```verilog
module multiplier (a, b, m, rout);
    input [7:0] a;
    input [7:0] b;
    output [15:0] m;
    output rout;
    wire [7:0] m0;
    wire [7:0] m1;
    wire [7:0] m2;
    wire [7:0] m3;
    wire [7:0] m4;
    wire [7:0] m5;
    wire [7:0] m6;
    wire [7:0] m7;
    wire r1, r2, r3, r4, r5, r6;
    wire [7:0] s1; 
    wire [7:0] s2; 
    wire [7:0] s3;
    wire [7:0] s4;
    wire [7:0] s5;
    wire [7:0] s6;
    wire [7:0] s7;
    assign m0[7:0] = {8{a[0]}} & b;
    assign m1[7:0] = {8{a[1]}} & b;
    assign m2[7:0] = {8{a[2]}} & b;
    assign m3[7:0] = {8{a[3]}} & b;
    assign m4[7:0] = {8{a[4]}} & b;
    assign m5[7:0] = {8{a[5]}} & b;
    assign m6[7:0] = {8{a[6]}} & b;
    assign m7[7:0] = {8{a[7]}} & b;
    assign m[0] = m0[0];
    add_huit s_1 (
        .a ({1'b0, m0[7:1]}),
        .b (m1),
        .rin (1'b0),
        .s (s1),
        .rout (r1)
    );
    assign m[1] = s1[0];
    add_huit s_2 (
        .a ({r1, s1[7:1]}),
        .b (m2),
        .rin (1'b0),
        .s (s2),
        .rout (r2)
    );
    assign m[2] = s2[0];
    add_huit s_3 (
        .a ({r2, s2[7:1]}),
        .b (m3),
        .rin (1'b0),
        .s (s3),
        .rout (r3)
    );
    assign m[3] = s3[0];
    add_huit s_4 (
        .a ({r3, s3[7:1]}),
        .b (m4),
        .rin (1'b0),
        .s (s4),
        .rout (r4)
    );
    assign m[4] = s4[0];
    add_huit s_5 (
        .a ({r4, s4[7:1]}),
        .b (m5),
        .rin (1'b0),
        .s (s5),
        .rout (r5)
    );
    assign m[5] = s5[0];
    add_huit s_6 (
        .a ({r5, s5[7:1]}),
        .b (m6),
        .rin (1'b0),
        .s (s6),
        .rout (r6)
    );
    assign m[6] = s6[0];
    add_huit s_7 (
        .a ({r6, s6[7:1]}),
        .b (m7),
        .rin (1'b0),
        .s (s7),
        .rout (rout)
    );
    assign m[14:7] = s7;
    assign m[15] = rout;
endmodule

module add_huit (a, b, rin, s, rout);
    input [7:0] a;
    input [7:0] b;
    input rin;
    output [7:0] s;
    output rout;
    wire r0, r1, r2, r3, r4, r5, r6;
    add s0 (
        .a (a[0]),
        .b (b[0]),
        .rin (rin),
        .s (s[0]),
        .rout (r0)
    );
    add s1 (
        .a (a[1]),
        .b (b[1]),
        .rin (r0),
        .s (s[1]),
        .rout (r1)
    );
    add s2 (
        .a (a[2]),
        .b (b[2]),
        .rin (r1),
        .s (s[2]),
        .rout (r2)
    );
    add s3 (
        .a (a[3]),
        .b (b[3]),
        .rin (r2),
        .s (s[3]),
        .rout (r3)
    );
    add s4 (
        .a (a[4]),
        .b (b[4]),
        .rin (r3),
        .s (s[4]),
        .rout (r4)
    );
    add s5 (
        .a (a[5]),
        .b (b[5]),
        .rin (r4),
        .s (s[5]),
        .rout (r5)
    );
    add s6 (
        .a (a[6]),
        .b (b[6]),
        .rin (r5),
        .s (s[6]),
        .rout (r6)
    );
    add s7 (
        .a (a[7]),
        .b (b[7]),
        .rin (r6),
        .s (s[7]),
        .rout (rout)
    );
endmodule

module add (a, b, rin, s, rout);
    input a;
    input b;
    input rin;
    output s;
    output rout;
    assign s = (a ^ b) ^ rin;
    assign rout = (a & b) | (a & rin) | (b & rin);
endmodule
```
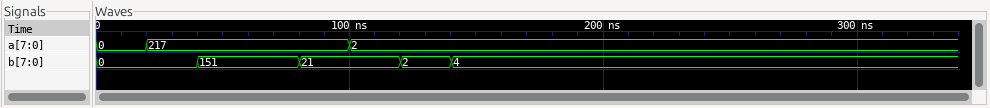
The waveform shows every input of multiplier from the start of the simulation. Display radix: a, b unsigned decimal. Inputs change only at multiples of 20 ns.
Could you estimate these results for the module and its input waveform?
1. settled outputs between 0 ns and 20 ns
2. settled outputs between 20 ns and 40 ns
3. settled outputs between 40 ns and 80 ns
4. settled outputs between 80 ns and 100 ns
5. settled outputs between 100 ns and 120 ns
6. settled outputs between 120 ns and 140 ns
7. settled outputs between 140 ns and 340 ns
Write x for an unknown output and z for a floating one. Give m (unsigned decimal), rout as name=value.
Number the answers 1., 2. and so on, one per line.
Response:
1. m=0, rout=0
2. m=0, rout=0
3. m=32767, rout=0
4. m=4557, rout=0
5. m=42, rout=0
6. m=4, rout=0
7. m=8, rout=0
